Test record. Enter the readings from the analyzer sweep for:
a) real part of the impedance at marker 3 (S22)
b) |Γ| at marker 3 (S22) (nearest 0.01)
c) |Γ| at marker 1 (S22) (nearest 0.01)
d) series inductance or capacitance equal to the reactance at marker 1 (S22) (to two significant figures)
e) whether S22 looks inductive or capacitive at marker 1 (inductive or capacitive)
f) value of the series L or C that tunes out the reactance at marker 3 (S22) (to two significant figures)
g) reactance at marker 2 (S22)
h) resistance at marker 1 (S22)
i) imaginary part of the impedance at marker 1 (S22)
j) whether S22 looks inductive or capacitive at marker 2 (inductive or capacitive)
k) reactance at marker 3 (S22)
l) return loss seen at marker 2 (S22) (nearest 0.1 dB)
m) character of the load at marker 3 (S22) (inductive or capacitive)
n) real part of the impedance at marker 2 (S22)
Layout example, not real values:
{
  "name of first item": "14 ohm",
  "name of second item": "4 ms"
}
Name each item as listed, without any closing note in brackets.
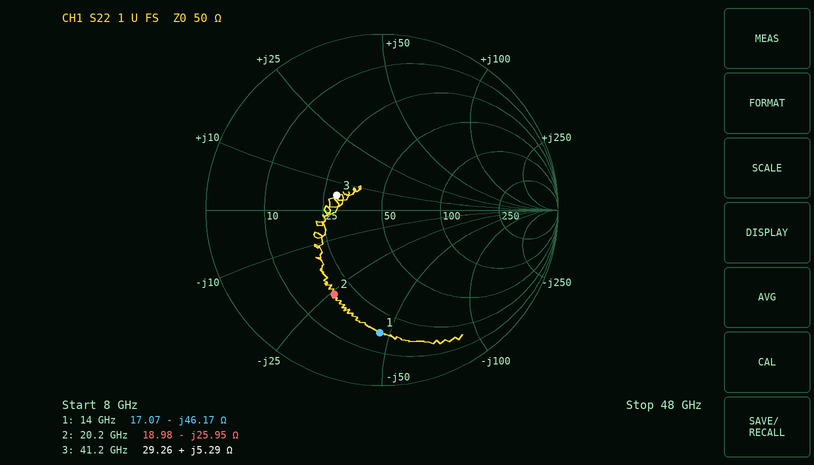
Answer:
{
  "real part of the impedance at marker 3": "29.26 Ω",
  "|Γ| at marker 3 (S22)": "0.27",
  "|Γ| at marker 1 (S22)": "0.70",
  "series inductance or capacitance equal to the reactance at marker 1 (S22)": "250 fF",
  "whether S22 looks inductive or capacitive at marker 1": "capacitive",
  "value of the series L or C that tunes out the reactance at marker 3 (S22)": "730 fF",
  "reactance at marker 2": "-25.95 Ω",
  "resistance at marker 1": "17.07 Ω",
  "imaginary part of the impedance at marker 1": "-46.17 Ω",
  "whether S22 looks inductive or capacitive at marker 2": "capacitive",
  "reactance at marker 3": "+5.29 Ω",
  "return loss seen at marker 2 (S22)": "5.2 dB",
  "character of the load at marker 3 (S22)": "inductive",
  "real part of the impedance at marker 2": "18.98 Ω"
}
